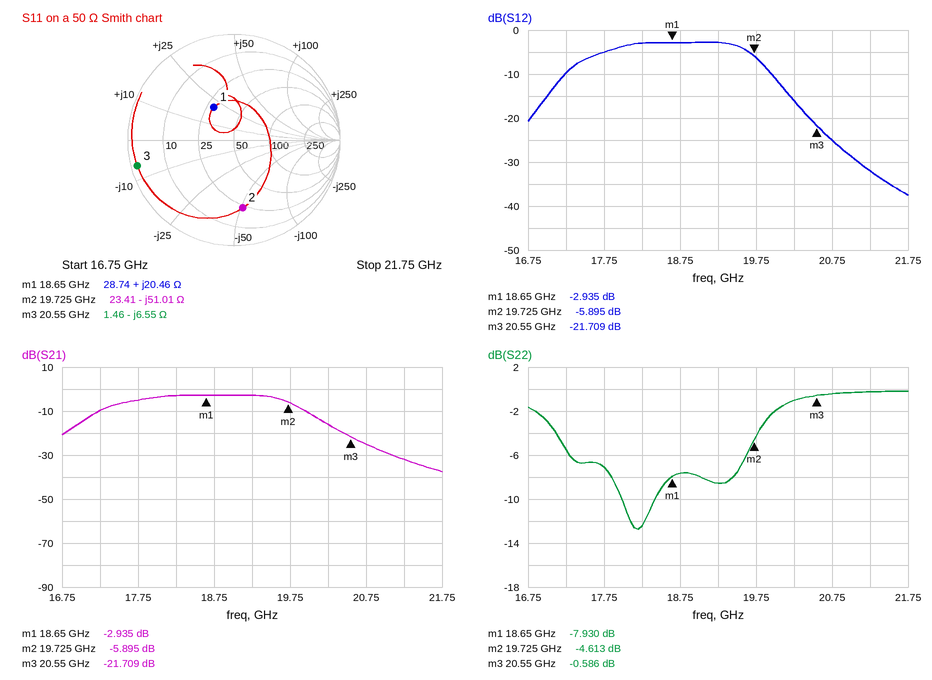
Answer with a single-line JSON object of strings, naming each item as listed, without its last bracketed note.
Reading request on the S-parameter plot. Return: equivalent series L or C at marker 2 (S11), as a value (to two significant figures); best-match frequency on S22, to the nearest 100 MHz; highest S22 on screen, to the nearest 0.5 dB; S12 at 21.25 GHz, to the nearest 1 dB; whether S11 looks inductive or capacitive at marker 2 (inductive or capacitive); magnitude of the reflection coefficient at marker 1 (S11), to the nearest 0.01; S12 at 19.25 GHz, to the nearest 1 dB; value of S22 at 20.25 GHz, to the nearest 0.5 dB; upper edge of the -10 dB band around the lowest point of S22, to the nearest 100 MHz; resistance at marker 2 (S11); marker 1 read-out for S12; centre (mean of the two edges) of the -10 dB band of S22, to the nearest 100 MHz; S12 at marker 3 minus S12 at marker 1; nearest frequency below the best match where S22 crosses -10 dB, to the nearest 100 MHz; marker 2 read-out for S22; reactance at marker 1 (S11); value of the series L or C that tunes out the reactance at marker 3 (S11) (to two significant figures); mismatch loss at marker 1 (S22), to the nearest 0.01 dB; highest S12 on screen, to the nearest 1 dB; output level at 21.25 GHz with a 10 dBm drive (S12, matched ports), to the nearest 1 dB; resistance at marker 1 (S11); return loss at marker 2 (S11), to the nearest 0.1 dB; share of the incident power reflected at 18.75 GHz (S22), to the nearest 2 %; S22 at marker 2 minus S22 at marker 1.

{"equivalent series L or C at marker 2 (S11), as a value": "160 fF", "best-match frequency on S22, to the nearest 100 MHz": "18.2 GHz", "highest S22 on screen, to the nearest 0.5 dB": "0.0 dB", "S12 at 21.25 GHz, to the nearest 1 dB": "-32 dB", "whether S11 looks inductive or capacitive at marker 2": "capacitive", "magnitude of the reflection coefficient at marker 1 (S11), to the nearest 0.01": "0.36", "S12 at 19.25 GHz, to the nearest 1 dB": "-3 dB", "value of S22 at 20.25 GHz, to the nearest 0.5 dB": "-1.0 dB", "upper edge of the -10 dB band around the lowest point of S22, to the nearest 100 MHz": "18.4 GHz", "resistance at marker 2": "23.41 Ω", "marker 1 read-out for S12": "-2.935 dB", "centre (mean of the two edges) of the -10 dB band of S22, to the nearest 100 MHz": "18.2 GHz", "S12 at marker 3 minus S12 at marker 1": "-18.774 dB", "nearest frequency below the best match where S22 crosses -10 dB, to the nearest 100 MHz": "18.0 GHz", "marker 2 read-out for S22": "-4.613 dB", "reactance at marker 1": "+20.46 Ω", "value of the series L or C that tunes out the reactance at marker 3 (S11)": "51 pH", "mismatch loss at marker 1 (S22), to the nearest 0.01 dB": "0.76 dB", "highest S12 on screen, to the nearest 1 dB": "-3 dB", "output level at 21.25 GHz with a 10 dBm drive (S12, matched ports), to the nearest 1 dB": "-22 dBm", "resistance at marker 1": "28.74 Ω", "return loss at marker 2 (S11), to the nearest 0.1 dB": "3.8 dB", "share of the incident power reflected at 18.75 GHz (S22), to the nearest 2 %": "18 %", "S22 at marker 2 minus S22 at marker 1": "3.317 dB"}
